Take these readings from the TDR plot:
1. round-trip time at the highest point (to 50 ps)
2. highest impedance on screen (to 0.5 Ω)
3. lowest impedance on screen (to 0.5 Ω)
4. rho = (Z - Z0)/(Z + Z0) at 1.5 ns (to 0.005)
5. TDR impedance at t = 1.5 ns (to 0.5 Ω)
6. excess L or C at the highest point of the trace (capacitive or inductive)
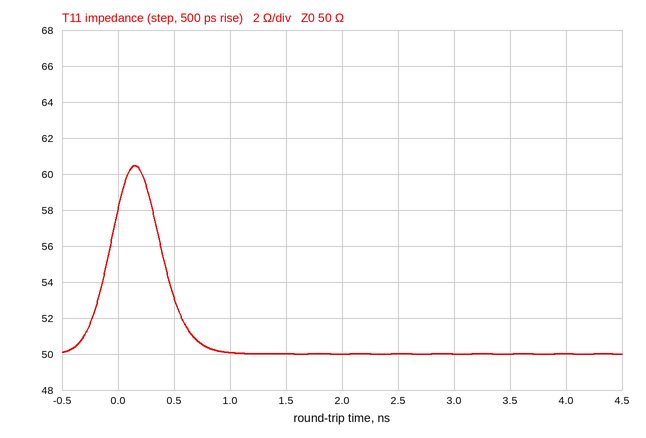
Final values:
150 ps
60.5 Ω
50.0 Ω
0.000
50.0 Ω
inductive
